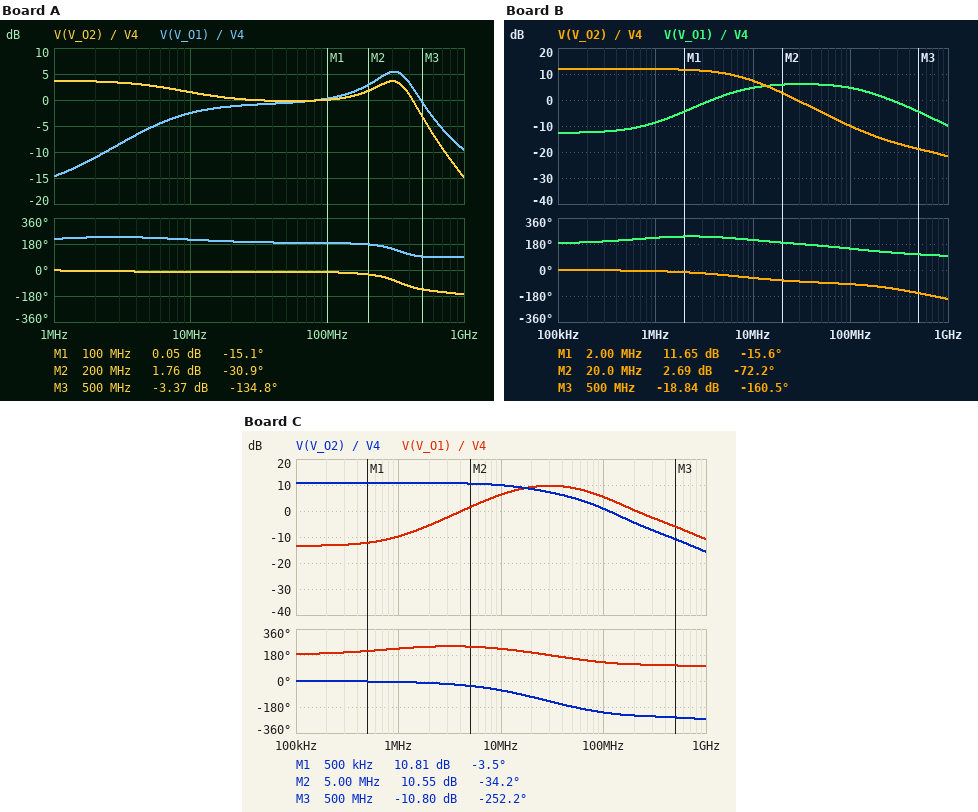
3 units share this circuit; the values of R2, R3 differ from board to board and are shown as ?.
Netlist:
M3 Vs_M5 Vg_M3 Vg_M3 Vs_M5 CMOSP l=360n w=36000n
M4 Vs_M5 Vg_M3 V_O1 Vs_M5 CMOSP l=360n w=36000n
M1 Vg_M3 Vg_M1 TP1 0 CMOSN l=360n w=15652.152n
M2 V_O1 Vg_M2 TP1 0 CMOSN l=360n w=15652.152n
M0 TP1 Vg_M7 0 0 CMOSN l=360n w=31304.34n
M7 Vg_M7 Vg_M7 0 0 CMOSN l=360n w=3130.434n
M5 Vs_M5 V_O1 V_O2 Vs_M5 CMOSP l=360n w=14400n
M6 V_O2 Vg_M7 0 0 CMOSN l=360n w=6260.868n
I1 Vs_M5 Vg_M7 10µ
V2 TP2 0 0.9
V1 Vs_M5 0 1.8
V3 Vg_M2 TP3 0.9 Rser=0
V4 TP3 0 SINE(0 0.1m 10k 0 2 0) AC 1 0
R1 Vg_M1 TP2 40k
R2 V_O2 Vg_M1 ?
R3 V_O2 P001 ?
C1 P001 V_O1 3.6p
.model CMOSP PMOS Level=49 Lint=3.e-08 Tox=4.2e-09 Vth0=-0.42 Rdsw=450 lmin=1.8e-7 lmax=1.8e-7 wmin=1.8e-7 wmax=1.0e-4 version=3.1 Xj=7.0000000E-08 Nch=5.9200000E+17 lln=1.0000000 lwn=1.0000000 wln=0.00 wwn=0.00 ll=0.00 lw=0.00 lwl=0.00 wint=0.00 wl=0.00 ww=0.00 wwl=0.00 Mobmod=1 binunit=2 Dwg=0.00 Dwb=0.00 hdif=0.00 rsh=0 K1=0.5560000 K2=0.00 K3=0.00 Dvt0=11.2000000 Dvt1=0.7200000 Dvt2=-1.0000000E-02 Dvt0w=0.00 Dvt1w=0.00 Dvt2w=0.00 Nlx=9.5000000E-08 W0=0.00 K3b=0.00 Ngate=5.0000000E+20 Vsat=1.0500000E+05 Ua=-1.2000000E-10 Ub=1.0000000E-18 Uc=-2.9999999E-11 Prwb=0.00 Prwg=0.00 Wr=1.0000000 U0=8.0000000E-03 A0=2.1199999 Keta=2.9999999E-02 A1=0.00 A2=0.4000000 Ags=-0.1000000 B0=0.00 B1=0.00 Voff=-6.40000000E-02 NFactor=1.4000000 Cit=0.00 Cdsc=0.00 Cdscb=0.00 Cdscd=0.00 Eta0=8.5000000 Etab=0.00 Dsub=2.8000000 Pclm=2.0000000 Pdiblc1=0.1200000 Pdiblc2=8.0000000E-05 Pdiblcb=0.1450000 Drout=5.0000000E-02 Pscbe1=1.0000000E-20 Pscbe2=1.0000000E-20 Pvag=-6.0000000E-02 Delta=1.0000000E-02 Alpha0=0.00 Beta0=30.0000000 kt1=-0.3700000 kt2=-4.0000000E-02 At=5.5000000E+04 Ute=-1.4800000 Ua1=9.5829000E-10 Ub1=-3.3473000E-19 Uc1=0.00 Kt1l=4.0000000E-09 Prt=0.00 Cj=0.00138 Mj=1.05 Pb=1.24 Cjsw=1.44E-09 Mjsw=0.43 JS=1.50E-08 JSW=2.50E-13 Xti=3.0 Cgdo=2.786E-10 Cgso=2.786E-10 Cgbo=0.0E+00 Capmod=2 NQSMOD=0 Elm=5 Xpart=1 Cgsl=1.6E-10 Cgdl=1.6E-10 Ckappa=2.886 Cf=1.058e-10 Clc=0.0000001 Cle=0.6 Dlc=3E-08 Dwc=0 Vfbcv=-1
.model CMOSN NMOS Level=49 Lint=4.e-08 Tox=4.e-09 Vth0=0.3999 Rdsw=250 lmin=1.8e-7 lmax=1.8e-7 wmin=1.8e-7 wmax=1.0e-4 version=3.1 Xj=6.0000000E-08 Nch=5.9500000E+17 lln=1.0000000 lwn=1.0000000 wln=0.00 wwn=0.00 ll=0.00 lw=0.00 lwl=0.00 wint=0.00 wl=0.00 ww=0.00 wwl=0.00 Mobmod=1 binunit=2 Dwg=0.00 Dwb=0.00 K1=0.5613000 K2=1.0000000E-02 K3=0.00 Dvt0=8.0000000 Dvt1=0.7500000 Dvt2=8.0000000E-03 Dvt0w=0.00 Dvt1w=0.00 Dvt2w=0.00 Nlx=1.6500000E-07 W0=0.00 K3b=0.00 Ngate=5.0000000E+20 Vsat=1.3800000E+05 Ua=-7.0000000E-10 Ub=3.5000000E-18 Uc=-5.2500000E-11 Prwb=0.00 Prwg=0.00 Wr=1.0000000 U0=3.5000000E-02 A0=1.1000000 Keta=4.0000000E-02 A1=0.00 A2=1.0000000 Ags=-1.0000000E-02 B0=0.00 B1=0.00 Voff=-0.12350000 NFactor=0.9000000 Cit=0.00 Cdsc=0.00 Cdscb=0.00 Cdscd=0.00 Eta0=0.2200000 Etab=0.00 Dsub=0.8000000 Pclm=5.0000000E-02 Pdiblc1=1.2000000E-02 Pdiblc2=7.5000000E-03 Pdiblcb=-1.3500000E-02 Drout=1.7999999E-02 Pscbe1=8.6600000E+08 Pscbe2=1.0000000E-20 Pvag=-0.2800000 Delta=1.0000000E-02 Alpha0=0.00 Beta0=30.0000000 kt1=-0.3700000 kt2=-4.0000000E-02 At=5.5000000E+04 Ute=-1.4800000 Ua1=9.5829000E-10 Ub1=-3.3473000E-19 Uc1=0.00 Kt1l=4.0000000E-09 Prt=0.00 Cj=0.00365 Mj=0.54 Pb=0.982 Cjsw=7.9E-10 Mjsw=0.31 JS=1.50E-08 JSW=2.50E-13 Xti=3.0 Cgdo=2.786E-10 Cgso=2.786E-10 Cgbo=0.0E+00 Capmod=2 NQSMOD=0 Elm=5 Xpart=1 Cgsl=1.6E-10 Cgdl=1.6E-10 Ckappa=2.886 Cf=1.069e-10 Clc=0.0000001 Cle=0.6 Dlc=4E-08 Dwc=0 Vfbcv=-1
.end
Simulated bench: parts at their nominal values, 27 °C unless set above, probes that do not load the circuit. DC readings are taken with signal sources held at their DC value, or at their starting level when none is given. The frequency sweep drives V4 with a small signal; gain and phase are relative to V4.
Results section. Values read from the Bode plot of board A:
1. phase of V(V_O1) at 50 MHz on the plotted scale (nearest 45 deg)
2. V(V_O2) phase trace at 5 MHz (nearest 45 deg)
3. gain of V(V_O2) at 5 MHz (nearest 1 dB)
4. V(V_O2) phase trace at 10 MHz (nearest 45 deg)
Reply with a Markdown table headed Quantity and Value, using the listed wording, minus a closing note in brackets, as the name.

| Quantity | Value |
|---|---|
| phase of V(V_O1) at 50 MHz on the plotted scale | 180 deg |
| V(V_O2) phase trace at 5 MHz | 0 deg |
| gain of V(V_O2) at 5 MHz | 3 dB |
| V(V_O2) phase trace at 10 MHz | 0 deg |
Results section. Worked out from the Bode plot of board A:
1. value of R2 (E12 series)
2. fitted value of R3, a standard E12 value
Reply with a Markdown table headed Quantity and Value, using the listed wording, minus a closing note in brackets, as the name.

| Quantity | Value |
|---|---|
| value of R2 | 22 kΩ |
| fitted value of R3, a standard E12 value | 6.8 kΩ |
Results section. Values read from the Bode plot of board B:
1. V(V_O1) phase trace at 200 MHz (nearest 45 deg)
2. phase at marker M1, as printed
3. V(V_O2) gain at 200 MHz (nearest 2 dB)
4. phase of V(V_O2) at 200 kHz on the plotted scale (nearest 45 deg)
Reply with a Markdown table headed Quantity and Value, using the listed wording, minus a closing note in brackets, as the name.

| Quantity | Value |
|---|---|
| V(V_O1) phase trace at 200 MHz | 135 deg |
| phase at marker M1, as printed | -15.6 deg |
| V(V_O2) gain at 200 MHz | -14 dB |
| phase of V(V_O2) at 200 kHz on the plotted scale | 0 deg |
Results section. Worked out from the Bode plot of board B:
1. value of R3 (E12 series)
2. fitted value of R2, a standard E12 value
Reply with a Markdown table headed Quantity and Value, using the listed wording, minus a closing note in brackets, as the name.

| Quantity | Value |
|---|---|
| value of R3 | 3.3 kΩ |
| fitted value of R2, a standard E12 value | 120 kΩ |
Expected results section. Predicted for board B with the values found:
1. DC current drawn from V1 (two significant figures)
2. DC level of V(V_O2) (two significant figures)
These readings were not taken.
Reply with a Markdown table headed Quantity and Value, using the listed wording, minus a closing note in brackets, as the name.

| Quantity | Value |
|---|---|
| DC current drawn from V1 | 120 µA |
| DC level of V(V_O2) | 900 mV |
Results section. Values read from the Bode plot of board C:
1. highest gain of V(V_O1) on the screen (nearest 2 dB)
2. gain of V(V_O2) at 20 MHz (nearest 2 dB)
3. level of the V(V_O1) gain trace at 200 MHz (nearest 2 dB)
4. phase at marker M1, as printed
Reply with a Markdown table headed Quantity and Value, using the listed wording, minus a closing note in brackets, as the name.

| Quantity | Value |
|---|---|
| highest gain of V(V_O1) on the screen | 10 dB |
| gain of V(V_O2) at 20 MHz | 8 dB |
| level of the V(V_O1) gain trace at 200 MHz | 0 dB |
| phase at marker M1, as printed | -3.5 deg |
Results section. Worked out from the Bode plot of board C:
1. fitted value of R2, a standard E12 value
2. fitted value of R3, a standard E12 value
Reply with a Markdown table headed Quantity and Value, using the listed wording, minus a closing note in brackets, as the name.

| Quantity | Value |
|---|---|
| fitted value of R2, a standard E12 value | 100 kΩ |
| fitted value of R3, a standard E12 value | 1.2 kΩ |
